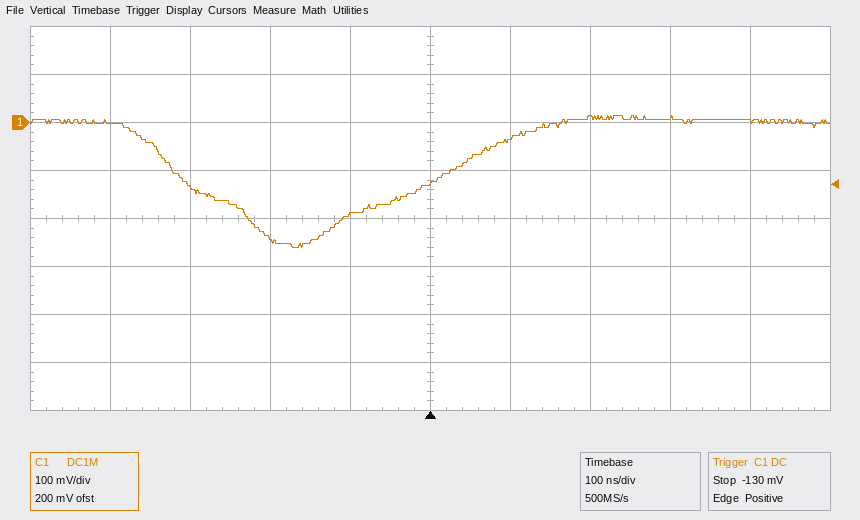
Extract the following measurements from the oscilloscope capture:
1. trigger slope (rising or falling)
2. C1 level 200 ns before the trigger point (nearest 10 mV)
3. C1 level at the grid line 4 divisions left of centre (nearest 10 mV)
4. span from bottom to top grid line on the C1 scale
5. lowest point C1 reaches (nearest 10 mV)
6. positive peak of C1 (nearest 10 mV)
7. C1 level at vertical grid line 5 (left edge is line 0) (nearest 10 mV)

rising
-240 mV
0 mV
800 mV
-260 mV
10 mV
-130 mV
